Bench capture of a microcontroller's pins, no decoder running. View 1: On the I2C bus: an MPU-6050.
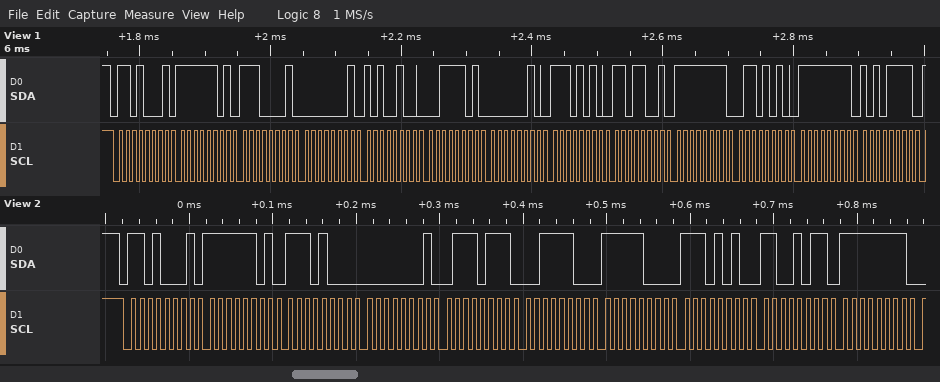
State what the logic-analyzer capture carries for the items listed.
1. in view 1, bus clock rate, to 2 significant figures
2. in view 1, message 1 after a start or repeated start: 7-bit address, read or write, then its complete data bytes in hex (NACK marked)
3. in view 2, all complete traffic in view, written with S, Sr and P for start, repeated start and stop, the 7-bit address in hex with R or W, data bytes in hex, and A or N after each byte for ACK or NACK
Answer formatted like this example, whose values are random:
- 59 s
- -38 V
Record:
- 100 kHz
- 0x68 read: FD E1 01 A4 3D 02 EA D9 FF 6A FF AF
- S 68R A FD A E8 A 01 A 77 A 3C A F8 A EA A CB A FF A
